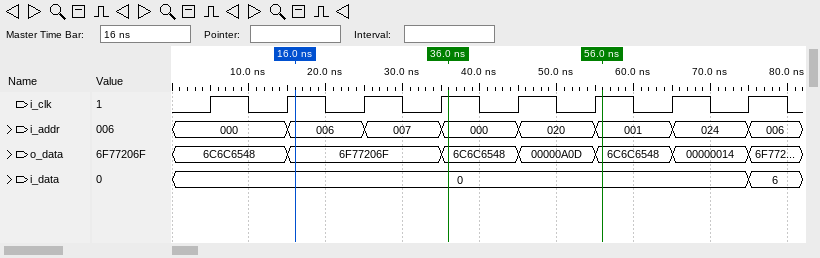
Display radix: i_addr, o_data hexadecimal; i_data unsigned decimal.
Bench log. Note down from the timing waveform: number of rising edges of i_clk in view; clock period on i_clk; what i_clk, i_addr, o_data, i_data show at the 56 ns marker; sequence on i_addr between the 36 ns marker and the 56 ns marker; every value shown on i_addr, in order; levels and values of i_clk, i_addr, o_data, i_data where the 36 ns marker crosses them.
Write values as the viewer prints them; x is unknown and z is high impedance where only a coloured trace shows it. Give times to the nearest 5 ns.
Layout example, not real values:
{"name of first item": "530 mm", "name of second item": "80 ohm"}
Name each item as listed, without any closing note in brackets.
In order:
{"number of rising edges of i_clk in view": "8", "clock period on i_clk": "10 ns", "what i_clk, i_addr, o_data, i_data show at the 56 ns marker": "i_clk=1, i_addr=001, o_data=6C6C6548, i_data=0", "sequence on i_addr between the 36 ns marker and the 56 ns marker": "000, 020, 001", "every value shown on i_addr, in order": "000, 006, 007, 000, 020, 001, 024, 006", "levels and values of i_clk, i_addr, o_data, i_data where the 36 ns marker crosses them": "i_clk=1, i_addr=000, o_data=6C6C6548, i_data=0"}
